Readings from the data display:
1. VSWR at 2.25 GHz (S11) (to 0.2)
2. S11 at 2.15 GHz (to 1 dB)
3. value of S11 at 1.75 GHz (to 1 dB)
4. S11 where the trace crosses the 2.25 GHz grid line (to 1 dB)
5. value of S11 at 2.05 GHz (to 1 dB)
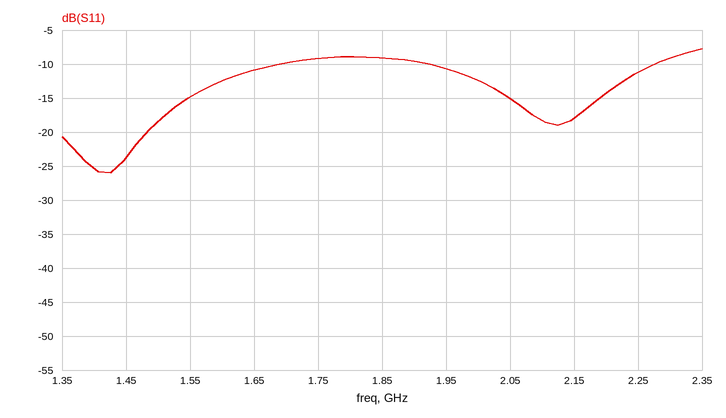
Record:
1.8
-18 dB
-9 dB
-11 dB
-15 dB
